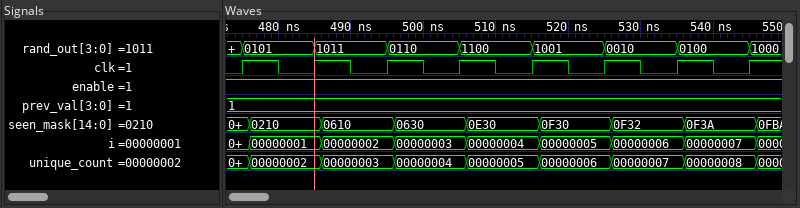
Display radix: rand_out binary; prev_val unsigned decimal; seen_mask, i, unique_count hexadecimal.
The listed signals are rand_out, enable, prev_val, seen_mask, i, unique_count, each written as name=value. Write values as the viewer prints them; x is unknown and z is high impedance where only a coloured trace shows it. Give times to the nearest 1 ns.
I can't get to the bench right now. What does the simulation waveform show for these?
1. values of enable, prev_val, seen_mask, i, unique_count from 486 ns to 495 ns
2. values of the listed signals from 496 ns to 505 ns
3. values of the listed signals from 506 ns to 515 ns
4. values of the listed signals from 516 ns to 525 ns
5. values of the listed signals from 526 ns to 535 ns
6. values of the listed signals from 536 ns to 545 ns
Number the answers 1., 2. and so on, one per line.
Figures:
1. enable=1, prev_val=1, seen_mask=0610, i=00000002, unique_count=00000003
2. rand_out=0110, enable=1, prev_val=1, seen_mask=0630, i=00000003, unique_count=00000004
3. rand_out=1100, enable=1, prev_val=1, seen_mask=0E30, i=00000004, unique_count=00000005
4. rand_out=1001, enable=1, prev_val=1, seen_mask=0F30, i=00000005, unique_count=00000006
5. rand_out=0010, enable=1, prev_val=1, seen_mask=0F32, i=00000006, unique_count=00000007
6. rand_out=0100, enable=1, prev_val=1, seen_mask=0F3A, i=00000007, unique_count=00000008
